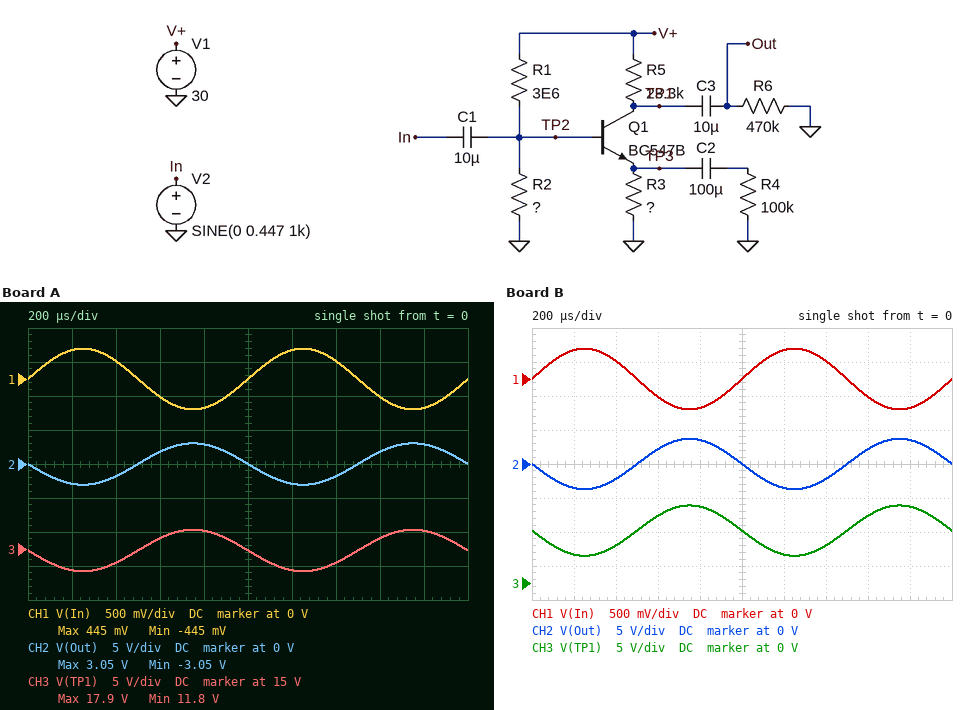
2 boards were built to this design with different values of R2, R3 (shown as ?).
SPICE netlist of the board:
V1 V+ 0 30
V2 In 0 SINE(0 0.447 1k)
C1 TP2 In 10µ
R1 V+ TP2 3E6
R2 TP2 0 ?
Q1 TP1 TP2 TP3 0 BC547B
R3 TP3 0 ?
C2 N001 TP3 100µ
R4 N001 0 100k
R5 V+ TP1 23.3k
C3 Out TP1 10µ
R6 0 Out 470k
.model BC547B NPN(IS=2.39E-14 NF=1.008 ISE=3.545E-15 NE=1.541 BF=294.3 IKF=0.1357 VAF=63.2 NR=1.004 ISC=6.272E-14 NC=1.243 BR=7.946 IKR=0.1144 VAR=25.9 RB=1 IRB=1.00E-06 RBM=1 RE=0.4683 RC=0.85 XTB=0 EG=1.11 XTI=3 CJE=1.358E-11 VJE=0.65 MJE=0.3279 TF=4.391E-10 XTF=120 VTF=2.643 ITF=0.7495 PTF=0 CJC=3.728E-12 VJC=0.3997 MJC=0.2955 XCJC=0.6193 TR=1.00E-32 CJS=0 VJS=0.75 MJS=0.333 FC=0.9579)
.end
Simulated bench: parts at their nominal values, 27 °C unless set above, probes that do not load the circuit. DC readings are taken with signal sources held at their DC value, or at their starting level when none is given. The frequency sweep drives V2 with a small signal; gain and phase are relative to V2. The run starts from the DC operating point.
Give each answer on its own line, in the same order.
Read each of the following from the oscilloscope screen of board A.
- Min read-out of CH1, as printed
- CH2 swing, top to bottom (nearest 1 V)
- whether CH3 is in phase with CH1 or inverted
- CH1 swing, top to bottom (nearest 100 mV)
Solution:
-445 mV
6 V
inverted
900 mV
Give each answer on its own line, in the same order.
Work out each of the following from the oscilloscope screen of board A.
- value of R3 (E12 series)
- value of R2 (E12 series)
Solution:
3.3 kΩ
390 kΩ
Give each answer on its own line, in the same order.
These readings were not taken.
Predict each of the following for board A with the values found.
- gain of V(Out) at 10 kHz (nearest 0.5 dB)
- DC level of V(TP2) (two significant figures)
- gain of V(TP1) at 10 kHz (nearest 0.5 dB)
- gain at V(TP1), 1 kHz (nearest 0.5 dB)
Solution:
16.5 dB
2.8 V
16.5 dB
16.5 dB
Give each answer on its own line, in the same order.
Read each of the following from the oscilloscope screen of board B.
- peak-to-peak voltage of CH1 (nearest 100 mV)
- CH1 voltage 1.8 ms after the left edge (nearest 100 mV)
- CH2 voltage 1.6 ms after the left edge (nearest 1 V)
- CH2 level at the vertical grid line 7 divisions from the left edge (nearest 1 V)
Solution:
900 mV
-400 mV
2 V
-2 V
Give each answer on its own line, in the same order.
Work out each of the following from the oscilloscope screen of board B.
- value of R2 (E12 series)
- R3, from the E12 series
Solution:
560 kΩ
2.7 kΩ
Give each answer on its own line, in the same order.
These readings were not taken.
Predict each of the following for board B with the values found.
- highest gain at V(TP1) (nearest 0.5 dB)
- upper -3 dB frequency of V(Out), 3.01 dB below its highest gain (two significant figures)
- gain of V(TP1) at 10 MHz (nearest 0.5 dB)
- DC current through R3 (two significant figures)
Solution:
18.5 dB
4.1 MHz
10.5 dB
960 µA
